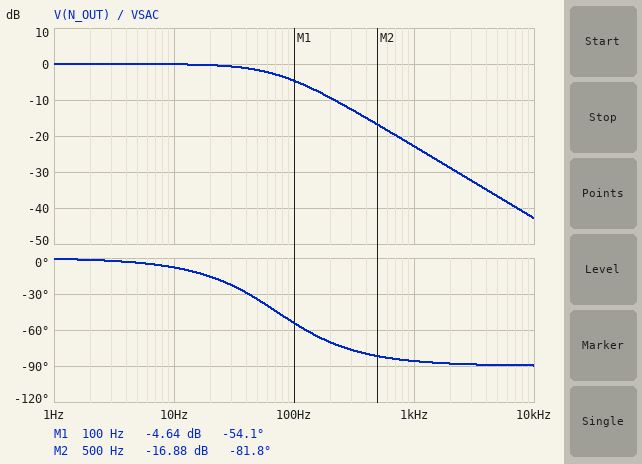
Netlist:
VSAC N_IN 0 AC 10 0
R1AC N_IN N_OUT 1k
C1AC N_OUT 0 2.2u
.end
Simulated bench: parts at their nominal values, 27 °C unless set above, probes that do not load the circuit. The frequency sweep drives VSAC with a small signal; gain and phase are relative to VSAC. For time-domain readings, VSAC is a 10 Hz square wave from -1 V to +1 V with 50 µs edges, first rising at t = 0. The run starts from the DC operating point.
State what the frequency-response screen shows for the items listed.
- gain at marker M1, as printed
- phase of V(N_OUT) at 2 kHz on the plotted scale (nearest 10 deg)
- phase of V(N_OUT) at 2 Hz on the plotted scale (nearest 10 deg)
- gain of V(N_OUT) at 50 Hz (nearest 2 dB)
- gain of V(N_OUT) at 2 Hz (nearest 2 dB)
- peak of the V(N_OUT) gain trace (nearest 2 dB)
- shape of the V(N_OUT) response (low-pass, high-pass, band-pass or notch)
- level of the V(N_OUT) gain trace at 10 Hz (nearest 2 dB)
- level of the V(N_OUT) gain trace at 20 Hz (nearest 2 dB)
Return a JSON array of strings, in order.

["-4.64 dB", "-90 deg", "0 deg", "-2 dB", "0 dB", "0 dB", "low-pass", "0 dB", "0 dB"]
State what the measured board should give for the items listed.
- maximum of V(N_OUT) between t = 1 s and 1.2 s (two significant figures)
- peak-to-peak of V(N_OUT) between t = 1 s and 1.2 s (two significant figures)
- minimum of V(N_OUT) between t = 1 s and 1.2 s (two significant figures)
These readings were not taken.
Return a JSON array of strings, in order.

["1.0 V", "2.0 V", "-1.0 V"]
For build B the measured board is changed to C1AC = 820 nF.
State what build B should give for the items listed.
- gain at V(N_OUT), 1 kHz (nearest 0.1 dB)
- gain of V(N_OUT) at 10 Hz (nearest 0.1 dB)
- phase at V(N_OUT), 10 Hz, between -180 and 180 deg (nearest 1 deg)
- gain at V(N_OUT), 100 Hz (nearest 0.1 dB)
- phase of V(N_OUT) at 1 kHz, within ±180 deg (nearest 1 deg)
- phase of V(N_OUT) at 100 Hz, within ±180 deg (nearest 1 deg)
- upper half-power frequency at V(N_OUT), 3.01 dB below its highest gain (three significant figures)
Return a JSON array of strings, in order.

["-14.4 dB", "0 dB", "-3 deg", "-1.0 dB", "-79 deg", "-27 deg", "194 Hz"]
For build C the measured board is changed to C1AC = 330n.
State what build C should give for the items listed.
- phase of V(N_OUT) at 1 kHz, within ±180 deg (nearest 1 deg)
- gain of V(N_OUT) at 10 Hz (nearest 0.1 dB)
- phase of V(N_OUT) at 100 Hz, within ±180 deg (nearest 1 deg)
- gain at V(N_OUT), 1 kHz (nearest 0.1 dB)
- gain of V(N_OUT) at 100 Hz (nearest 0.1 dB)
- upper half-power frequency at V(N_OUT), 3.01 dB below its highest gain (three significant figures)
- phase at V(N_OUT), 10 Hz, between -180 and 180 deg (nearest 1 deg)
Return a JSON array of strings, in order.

["-64 deg", "0 dB", "-12 deg", "-7.2 dB", "-0.2 dB", "482 Hz", "-1 deg"]
